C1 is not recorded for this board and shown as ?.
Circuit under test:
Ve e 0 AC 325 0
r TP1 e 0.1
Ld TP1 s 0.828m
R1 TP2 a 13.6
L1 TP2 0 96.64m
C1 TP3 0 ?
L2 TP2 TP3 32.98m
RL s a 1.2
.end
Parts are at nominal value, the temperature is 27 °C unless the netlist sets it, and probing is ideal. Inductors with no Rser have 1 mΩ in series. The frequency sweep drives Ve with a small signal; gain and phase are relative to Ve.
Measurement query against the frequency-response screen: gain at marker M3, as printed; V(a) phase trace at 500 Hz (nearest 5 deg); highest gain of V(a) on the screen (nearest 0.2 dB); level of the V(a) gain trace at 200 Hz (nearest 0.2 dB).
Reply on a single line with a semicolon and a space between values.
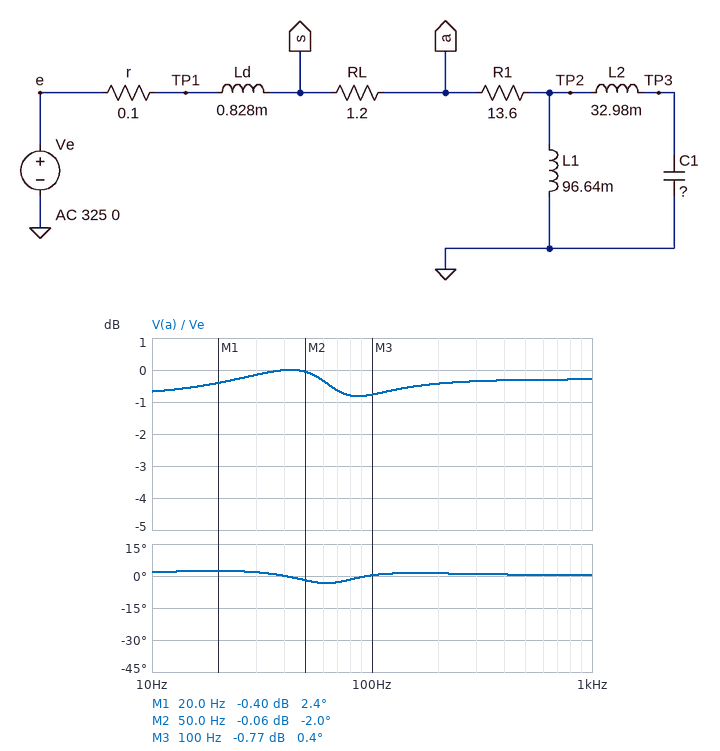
-0.77 dB; 0 deg; 0 dB; -0.4 dB
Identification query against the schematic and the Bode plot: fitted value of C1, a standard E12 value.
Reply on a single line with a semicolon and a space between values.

120 µF
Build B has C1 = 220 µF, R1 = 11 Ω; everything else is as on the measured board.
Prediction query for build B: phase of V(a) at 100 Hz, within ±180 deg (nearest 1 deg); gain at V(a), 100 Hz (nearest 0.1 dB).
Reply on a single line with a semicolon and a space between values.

2 deg; -0.7 dB
